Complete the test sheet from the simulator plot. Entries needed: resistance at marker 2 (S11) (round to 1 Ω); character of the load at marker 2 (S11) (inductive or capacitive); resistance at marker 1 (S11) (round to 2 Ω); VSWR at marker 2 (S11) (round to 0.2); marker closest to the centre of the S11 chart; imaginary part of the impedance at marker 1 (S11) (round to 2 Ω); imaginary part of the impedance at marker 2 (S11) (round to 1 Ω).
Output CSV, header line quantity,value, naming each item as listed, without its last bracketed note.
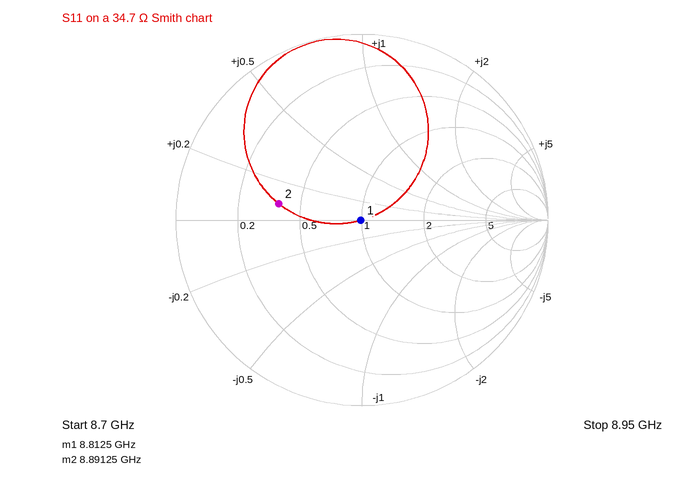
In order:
quantity,value
resistance at marker 2 (S11),13 Ω
character of the load at marker 2 (S11),inductive
resistance at marker 1 (S11),34 Ω
VSWR at marker 2 (S11),2.6
marker closest to the centre of the S11 chart,marker 1
imaginary part of the impedance at marker 1 (S11),0 Ω
imaginary part of the impedance at marker 2 (S11),+3 Ω
